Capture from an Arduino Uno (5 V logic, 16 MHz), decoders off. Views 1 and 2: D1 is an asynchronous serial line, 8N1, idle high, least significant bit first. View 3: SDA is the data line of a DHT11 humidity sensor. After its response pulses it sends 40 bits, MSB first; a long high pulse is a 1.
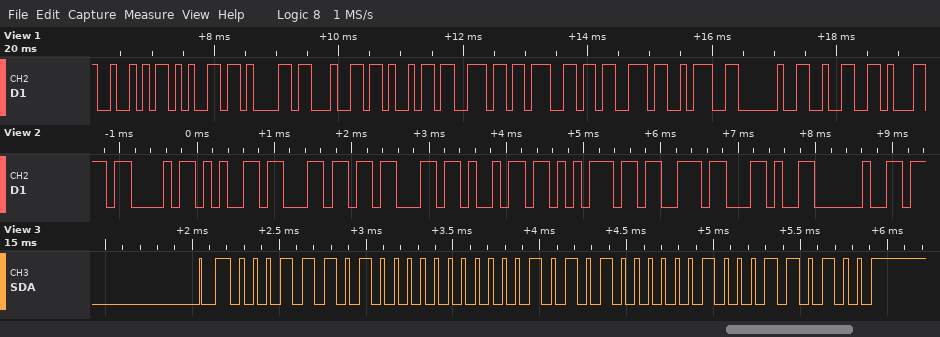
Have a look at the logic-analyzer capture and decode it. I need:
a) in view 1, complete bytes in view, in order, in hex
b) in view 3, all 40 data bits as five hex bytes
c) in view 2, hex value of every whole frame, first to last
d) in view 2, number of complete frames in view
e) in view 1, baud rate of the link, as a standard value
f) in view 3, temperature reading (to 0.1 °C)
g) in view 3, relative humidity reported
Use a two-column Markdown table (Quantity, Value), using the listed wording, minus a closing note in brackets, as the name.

| Quantity | Value |
|---|---|
| in view 1, complete bytes in view, in order, in hex | 0x52 0x65 0x61 0x64 0x69 0x6E 0x67 0x73 0x3A 0x20 0x32 |
| in view 3, all 40 data bits as five hex bytes | 1D 00 15 02 34 |
| in view 2, hex value of every whole frame, first to last | 43 65 6C 63 69 75 73 2C 20 |
| in view 2, number of complete frames in view | 9 |
| in view 1, baud rate of the link, as a standard value | 9600 baud |
| in view 3, temperature reading | 21.2 °C |
| in view 3, relative humidity reported | 29 % |
